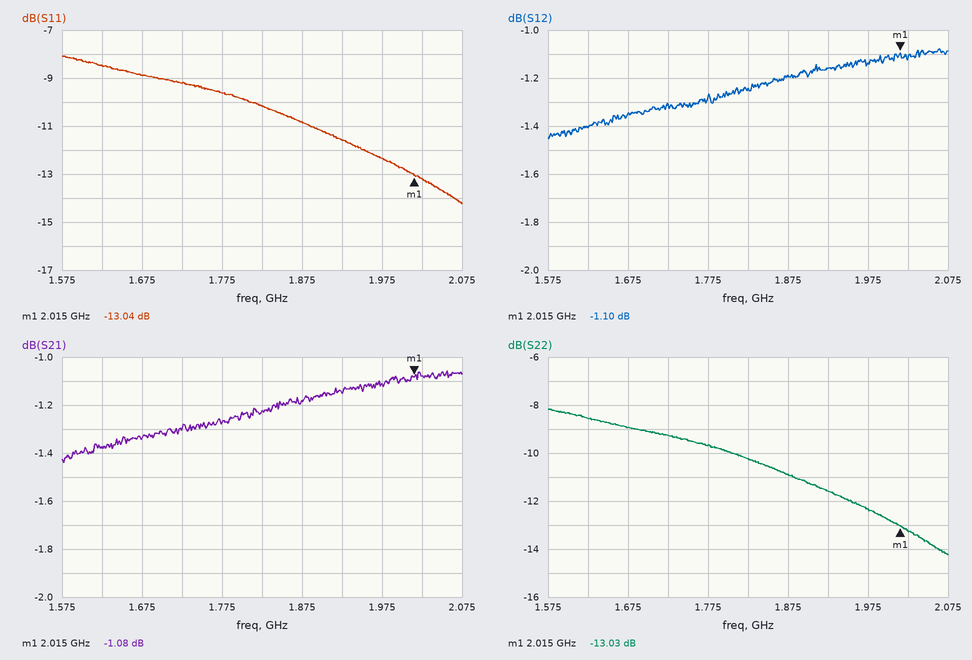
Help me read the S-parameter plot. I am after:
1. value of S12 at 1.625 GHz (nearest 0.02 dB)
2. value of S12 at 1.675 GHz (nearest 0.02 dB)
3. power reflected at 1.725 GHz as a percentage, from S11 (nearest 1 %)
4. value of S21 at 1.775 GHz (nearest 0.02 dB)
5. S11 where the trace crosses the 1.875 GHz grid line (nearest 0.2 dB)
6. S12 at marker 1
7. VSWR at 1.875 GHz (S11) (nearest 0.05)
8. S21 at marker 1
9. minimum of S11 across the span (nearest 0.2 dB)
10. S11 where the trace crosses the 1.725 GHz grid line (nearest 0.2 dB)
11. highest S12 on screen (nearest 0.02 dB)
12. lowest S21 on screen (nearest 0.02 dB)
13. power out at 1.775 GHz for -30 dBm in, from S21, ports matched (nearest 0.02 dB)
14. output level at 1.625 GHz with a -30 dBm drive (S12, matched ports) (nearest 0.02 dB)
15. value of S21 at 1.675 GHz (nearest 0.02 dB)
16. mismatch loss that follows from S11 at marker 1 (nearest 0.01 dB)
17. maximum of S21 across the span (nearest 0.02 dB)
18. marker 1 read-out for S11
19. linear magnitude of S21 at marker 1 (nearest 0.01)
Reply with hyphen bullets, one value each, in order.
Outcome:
- -1.40 dB
- -1.34 dB
- 12 %
- -1.28 dB
- -10.8 dB
- -1.10 dB
- 1.80
- -1.08 dB
- -14.2 dB
- -9.2 dB
- -1.08 dB
- -1.44 dB
- -31.28 dBm
- -31.40 dBm
- -1.34 dB
- 0.22 dB
- -1.06 dB
- -13.04 dB
- 0.88
